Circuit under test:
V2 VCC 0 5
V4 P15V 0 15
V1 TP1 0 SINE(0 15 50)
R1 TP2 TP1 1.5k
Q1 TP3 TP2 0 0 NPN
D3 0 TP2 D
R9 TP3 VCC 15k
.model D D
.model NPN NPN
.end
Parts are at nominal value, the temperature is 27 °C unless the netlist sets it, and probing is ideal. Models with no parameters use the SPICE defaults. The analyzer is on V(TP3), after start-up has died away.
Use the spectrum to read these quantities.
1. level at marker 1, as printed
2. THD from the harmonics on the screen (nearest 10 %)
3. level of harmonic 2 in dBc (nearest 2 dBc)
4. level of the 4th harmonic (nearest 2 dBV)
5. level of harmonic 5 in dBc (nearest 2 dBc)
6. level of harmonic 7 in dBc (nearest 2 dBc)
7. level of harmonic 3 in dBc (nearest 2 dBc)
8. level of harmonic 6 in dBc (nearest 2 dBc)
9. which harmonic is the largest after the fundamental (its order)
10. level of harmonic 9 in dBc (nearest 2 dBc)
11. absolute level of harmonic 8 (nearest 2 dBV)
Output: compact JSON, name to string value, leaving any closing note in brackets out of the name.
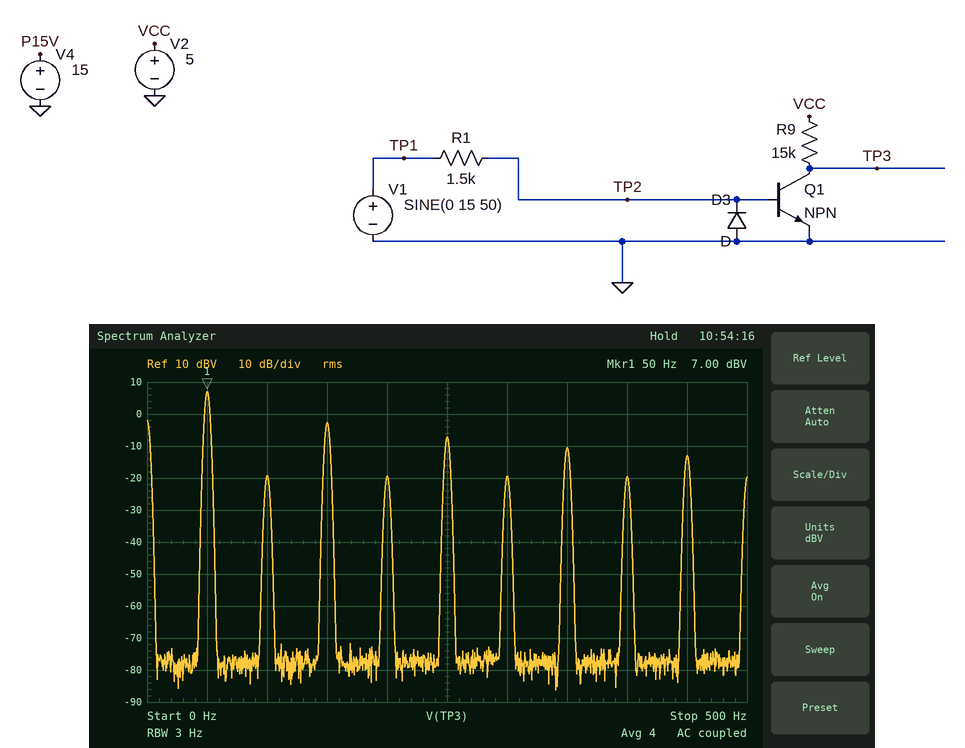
{"level at marker 1, as printed": "7.00 dBV", "THD from the harmonics on the screen": "40 %", "level of harmonic 2 in dBc": "-26 dBc", "level of the 4th harmonic": "-20 dBV", "level of harmonic 5 in dBc": "-14 dBc", "level of harmonic 7 in dBc": "-18 dBc", "level of harmonic 3 in dBc": "-10 dBc", "level of harmonic 6 in dBc": "-26 dBc", "which harmonic is the largest after the fundamental": "3", "level of harmonic 9 in dBc": "-20 dBc", "absolute level of harmonic 8": "-20 dBV"}
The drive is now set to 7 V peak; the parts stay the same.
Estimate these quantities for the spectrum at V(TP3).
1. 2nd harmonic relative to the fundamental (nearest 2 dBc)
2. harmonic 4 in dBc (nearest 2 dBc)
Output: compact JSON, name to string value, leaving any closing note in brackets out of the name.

{"2nd harmonic relative to the fundamental": "-20 dBc", "harmonic 4 in dBc": "-20 dBc"}
